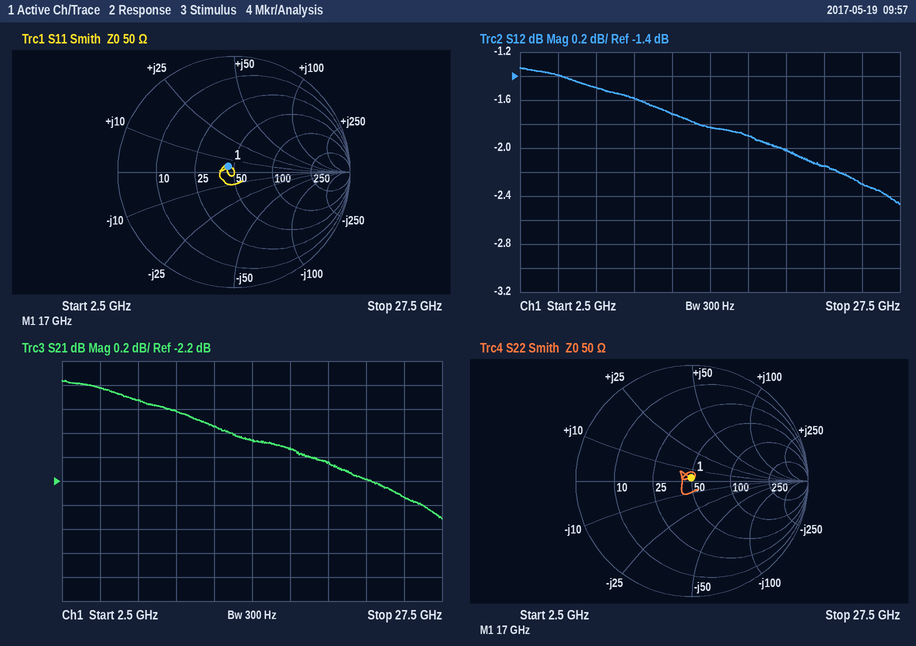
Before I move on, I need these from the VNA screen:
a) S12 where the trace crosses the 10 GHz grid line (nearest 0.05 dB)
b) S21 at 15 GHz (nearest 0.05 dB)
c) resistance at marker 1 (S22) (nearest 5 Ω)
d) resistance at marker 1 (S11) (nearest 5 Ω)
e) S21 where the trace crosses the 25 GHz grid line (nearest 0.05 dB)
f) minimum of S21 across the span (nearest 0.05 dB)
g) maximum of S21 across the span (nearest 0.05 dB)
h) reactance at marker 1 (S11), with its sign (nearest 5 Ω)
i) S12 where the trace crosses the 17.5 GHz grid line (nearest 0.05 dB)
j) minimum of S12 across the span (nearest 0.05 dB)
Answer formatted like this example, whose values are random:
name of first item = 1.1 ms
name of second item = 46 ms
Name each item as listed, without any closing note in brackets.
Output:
S12 where the trace crosses the 10 GHz grid line = -1.60 dB
S21 at 15 GHz = -1.85 dB
resistance at marker 1 (S22) = 50 Ω
resistance at marker 1 (S11) = 45 Ω
S21 where the trace crosses the 25 GHz grid line = -2.35 dB
minimum of S21 across the span = -2.50 dB
maximum of S21 across the span = -1.35 dB
reactance at marker 1 (S11), with its sign = +5 Ω
S12 where the trace crosses the 17.5 GHz grid line = -1.90 dB
minimum of S12 across the span = -2.45 dB
